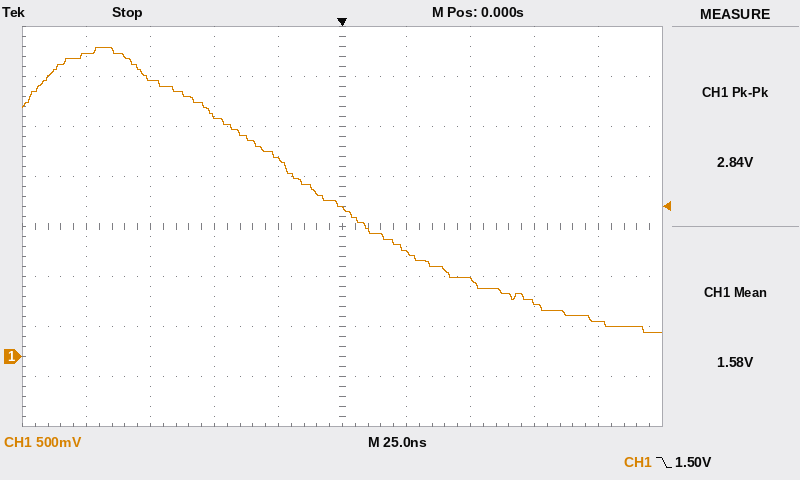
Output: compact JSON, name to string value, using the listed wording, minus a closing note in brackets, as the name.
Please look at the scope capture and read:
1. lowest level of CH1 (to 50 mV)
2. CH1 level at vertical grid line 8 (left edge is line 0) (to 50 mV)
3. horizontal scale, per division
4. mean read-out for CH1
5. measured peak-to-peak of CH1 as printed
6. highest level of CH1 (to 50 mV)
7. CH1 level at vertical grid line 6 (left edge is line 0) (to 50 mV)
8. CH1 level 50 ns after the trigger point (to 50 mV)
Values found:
{"lowest level of CH1": "250 mV", "CH1 level at vertical grid line 8 (left edge is line 0)": "550 mV", "horizontal scale, per division": "25 ns", "mean read-out for CH1": "1.58 V", "measured peak-to-peak of CH1 as printed": "2.84 V", "highest level of CH1": "3.10 V", "CH1 level at vertical grid line 6 (left edge is line 0)": "1.05 V", "CH1 level 50 ns after the trigger point": "750 mV"}
